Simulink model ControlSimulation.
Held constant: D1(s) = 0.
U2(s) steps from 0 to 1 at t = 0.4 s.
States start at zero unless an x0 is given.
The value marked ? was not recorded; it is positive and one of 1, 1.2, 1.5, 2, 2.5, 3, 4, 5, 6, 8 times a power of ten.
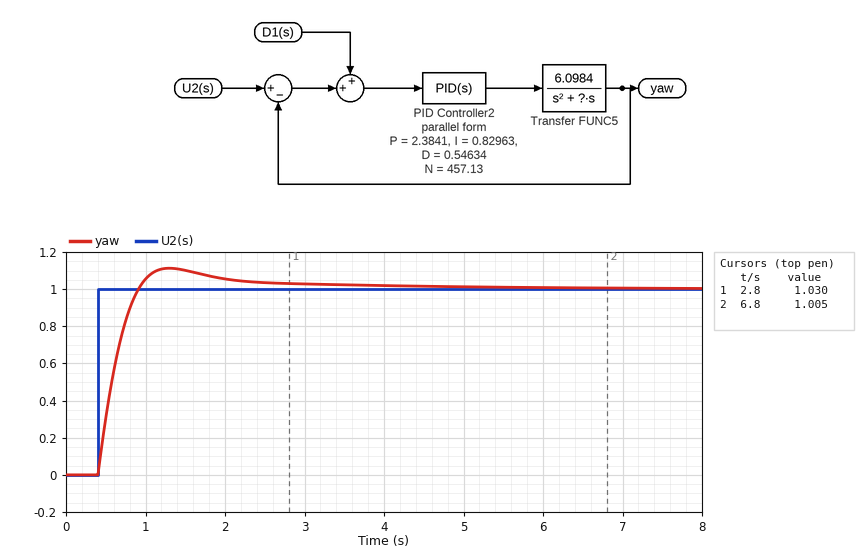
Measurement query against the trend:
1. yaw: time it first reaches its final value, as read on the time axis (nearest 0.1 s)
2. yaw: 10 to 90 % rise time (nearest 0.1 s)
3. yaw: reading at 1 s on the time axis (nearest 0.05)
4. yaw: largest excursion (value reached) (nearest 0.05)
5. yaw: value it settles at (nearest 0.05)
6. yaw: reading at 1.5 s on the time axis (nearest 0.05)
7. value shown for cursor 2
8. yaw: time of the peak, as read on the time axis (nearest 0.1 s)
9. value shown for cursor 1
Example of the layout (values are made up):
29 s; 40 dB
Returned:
0.9 s; 0.4 s; 1.05; 1.10; 1.00; 1.10; 1.005; 1.3 s; 1.030
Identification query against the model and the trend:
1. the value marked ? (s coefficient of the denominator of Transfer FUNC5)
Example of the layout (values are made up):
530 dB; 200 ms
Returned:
2.5
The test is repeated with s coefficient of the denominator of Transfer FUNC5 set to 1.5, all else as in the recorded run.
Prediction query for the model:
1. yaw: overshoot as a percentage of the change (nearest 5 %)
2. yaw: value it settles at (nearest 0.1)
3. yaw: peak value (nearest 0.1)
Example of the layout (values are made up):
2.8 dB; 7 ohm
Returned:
20 %; 1.0; 1.2
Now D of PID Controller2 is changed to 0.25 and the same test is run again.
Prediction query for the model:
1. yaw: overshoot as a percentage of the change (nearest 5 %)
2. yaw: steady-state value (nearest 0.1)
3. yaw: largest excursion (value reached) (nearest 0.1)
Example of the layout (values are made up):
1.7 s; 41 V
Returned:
25 %; 1.0; 1.2
